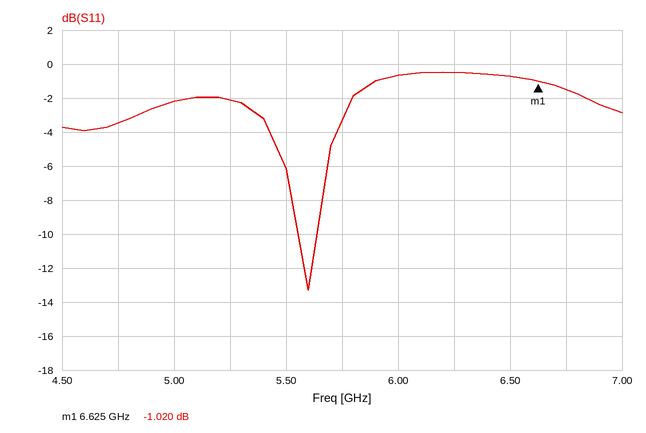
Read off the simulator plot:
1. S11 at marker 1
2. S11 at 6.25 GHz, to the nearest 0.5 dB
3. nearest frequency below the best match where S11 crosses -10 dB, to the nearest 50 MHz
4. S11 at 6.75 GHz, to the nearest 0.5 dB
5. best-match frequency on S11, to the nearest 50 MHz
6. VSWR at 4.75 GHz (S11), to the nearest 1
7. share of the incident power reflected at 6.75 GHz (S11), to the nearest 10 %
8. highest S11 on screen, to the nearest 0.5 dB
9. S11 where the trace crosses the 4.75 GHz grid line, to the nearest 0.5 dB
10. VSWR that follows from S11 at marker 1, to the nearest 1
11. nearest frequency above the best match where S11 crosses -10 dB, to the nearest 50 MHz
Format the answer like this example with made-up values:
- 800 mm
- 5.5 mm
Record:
- -1.020 dB
- -0.5 dB
- 5.55 GHz
- -1.5 dB
- 5.60 GHz
- 5
- 70 %
- -0.5 dB
- -3.5 dB
- 17
- 5.65 GHz
